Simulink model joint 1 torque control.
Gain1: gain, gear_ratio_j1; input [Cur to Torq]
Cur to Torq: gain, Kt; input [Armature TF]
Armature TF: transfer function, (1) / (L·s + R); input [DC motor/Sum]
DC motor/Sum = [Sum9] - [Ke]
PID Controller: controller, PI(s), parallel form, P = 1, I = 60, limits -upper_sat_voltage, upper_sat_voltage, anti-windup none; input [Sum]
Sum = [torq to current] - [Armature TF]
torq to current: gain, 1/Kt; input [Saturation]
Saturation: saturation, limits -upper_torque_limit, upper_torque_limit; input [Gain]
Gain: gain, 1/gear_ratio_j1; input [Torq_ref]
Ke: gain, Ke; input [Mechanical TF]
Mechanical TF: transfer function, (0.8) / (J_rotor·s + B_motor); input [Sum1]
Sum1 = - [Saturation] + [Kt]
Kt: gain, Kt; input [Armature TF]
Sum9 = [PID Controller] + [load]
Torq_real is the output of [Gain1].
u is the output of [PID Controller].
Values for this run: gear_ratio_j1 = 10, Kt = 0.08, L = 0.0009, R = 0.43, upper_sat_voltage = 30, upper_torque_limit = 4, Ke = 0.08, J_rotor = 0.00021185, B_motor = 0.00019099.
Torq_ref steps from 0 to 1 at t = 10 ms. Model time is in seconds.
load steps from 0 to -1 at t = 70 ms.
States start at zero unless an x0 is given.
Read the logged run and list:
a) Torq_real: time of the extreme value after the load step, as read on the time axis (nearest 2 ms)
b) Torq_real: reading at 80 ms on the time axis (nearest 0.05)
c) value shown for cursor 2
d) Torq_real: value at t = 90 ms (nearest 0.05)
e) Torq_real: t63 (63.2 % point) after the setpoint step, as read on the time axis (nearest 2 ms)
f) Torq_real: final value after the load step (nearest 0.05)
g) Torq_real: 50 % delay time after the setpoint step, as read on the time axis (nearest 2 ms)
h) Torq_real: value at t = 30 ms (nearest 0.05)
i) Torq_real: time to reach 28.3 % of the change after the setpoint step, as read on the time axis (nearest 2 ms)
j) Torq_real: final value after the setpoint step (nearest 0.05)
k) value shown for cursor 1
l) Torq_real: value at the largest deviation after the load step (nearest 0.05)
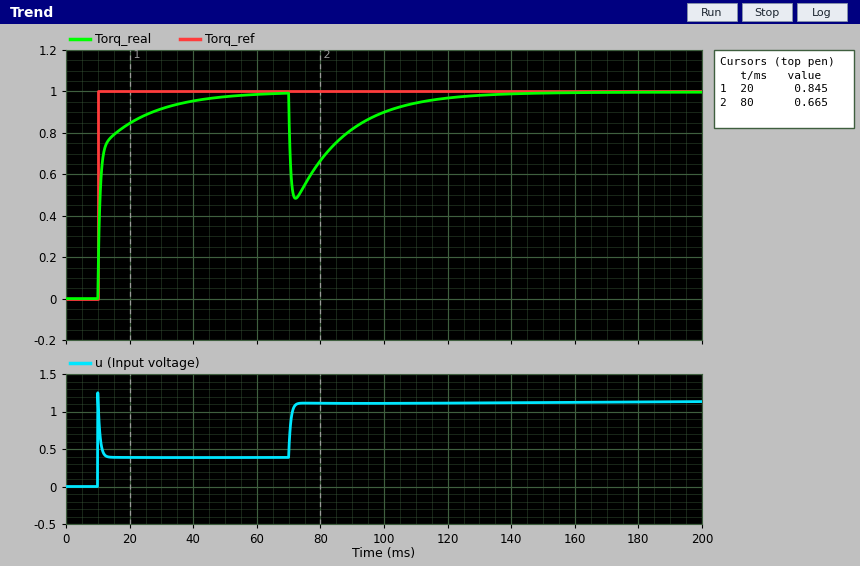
72 ms
0.65
0.665
0.80
12 ms
1.00
10 ms
0.90
10 ms
1.00
0.845
0.50
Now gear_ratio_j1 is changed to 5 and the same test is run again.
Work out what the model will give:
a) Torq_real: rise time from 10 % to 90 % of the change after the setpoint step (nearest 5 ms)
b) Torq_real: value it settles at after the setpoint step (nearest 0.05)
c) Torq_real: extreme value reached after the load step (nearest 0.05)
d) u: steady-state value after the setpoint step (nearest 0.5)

15 ms
1.00
0.75
1.0
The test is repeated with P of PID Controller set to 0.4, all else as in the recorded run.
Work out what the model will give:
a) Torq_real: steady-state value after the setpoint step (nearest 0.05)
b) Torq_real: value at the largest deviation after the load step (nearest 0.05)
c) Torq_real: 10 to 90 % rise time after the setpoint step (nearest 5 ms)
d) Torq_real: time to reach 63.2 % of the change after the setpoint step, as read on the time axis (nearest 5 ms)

1.00
0.20
15 ms
15 ms
